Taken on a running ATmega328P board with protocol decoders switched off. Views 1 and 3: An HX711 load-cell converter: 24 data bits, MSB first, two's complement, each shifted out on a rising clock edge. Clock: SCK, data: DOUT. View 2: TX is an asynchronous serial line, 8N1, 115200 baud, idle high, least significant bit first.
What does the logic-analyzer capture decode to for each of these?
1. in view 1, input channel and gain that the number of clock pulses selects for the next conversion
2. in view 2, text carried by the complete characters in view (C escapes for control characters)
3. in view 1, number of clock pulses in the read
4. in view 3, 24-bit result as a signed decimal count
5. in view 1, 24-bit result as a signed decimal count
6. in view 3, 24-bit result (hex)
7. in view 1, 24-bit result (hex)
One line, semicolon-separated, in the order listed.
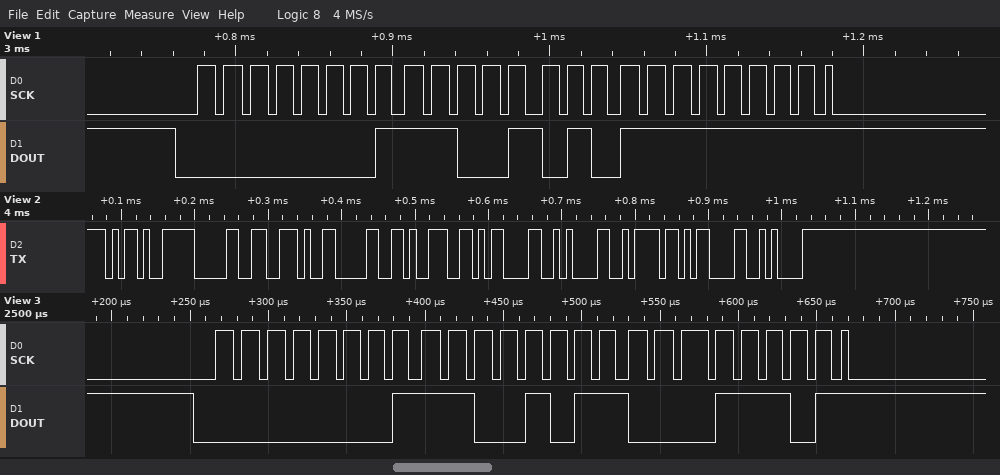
channel A, gain 128; "-0.09\r\nz\r\n"; 25; 117533; 117503; 0x01CB1D; 0x01CAFF
